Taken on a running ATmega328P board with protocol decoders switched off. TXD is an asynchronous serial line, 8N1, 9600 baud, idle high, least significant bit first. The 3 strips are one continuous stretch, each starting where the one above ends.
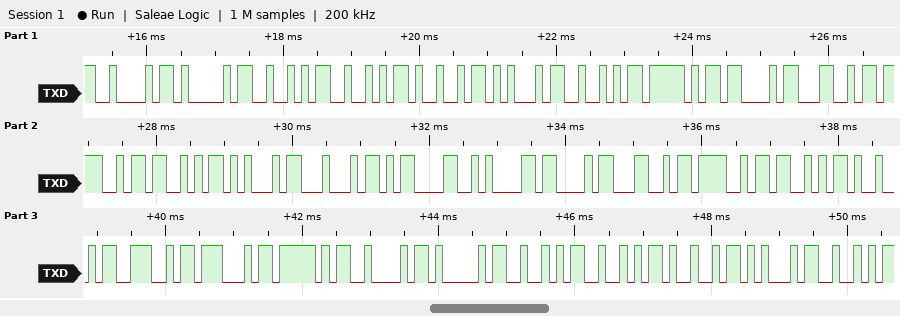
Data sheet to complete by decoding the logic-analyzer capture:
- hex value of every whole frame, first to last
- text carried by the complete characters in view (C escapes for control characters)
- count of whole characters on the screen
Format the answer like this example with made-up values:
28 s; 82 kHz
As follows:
42 41 52 52 49 45 52 5F 43 4C 4F 53 45 44 0D 0A 43 4C 4F 53 49 4E 47 5F 42 41 52 52 49 45 52; "BARRIER_CLOSED\r\nCLOSING_BARRIER"; 31
